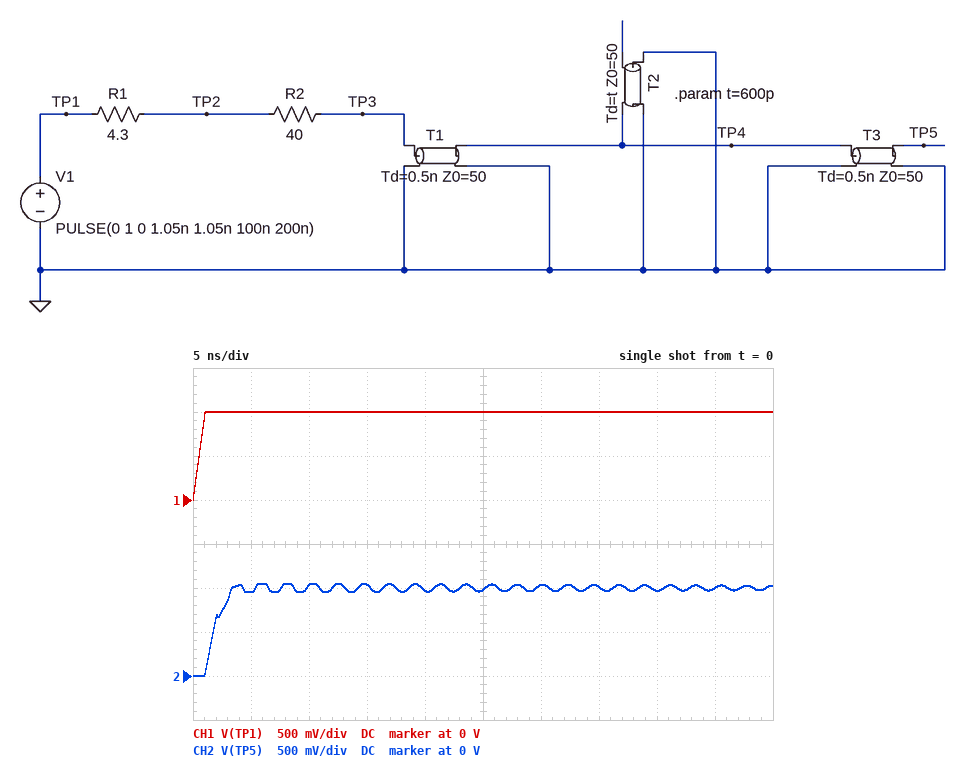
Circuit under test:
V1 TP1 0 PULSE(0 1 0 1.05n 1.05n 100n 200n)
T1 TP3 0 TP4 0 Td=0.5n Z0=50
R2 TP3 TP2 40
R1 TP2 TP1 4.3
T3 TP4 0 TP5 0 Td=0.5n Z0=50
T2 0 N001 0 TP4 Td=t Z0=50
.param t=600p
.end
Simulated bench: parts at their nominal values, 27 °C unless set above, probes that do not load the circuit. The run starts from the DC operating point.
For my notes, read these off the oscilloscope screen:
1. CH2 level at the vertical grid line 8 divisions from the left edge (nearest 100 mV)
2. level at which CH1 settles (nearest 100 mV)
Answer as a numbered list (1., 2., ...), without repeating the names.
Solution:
1. 1.0 V
2. 1.0 V
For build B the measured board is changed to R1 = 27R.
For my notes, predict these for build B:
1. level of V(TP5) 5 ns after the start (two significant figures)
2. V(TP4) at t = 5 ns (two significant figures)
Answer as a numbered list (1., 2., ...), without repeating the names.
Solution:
1. 850 mV
2. 890 mV
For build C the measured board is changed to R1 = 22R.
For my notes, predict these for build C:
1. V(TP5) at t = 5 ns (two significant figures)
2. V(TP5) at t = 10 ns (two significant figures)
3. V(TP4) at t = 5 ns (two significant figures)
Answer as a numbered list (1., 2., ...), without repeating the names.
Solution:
1. 880 mV
2. 1.0 V
3. 910 mV
